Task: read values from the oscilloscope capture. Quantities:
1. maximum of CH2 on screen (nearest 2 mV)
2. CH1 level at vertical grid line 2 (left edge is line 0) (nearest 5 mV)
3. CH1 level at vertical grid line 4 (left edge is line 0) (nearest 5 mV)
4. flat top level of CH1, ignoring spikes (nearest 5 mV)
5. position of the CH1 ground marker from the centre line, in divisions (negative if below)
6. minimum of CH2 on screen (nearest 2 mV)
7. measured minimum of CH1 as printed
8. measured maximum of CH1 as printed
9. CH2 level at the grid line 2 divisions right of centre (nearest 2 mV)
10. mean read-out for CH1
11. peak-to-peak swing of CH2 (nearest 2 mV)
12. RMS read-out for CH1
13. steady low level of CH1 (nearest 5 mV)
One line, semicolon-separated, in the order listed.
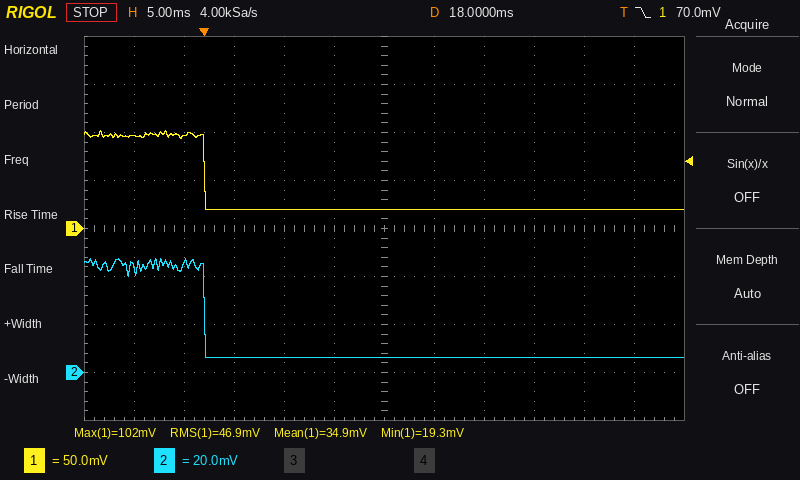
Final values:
48 mV; 95 mV; 20 mV; 95 mV; 0.0 div; 6 mV; 19.3 mV; 102 mV; 6 mV; 34.9 mV; 42 mV; 46.9 mV; 20 mV
